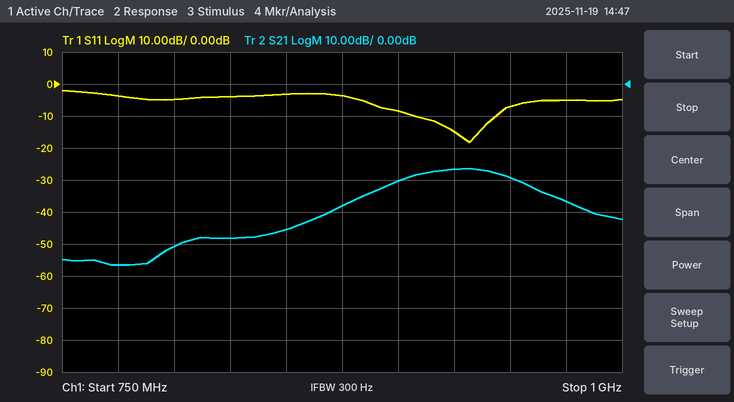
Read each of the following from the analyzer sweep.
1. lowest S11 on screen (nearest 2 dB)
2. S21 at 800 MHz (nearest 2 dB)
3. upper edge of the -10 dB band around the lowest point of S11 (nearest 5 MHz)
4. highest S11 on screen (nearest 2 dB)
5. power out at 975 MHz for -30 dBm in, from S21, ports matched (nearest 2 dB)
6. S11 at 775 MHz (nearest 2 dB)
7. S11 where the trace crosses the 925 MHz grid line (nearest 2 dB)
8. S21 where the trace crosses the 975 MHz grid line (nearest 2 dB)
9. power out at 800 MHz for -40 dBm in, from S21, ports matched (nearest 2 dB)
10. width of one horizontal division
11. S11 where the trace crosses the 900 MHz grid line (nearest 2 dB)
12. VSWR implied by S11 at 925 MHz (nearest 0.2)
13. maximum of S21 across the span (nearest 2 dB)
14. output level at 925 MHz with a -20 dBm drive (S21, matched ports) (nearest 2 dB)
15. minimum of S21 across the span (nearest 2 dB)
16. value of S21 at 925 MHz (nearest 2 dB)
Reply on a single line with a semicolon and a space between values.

-18 dB; -50 dB; 945 MHz; -2 dB; -66 dBm; -4 dB; -14 dB; -36 dB; -90 dBm; 25 MHz; -8 dB; 1.4; -26 dB; -46 dBm; -56 dB; -26 dB
